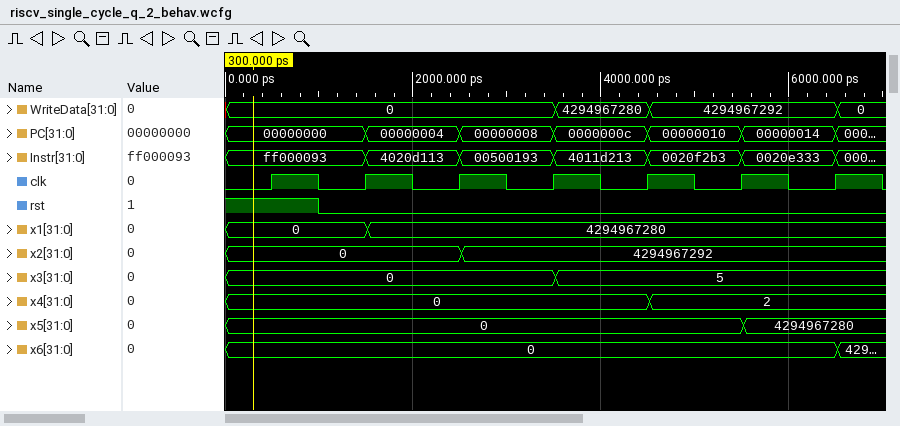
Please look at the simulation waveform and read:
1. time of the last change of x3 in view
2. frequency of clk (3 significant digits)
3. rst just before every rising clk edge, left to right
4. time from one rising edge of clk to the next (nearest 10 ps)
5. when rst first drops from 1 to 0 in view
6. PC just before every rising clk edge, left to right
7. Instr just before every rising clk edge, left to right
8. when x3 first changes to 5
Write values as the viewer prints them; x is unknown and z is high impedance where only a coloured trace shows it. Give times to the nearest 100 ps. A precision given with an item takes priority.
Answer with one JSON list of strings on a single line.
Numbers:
["3500 ps", "1.00 GHz", "1 0 0 0 0 0 0", "1000 ps", "1000 ps", "00000000, 00000000, 00000004, 00000008, 0000000c, 00000010, 00000014", "ff000093, ff000093, 4020d113, 00500193, 4011d213, 0020f2b3, 0020e333", "3500 ps"]
